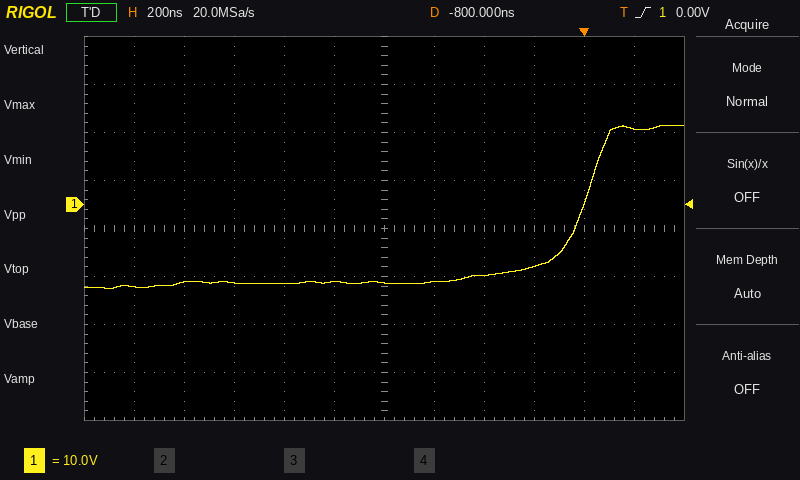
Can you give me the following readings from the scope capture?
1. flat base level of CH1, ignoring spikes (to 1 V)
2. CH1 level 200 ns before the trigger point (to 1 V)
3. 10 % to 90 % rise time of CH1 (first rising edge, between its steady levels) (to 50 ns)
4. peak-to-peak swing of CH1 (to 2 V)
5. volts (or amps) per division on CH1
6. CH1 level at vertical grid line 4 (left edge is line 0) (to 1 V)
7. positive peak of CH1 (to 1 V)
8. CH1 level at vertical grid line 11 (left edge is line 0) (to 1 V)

-16 V
-13 V
300 ns
34 V
10 V
-16 V
16 V
16 V
